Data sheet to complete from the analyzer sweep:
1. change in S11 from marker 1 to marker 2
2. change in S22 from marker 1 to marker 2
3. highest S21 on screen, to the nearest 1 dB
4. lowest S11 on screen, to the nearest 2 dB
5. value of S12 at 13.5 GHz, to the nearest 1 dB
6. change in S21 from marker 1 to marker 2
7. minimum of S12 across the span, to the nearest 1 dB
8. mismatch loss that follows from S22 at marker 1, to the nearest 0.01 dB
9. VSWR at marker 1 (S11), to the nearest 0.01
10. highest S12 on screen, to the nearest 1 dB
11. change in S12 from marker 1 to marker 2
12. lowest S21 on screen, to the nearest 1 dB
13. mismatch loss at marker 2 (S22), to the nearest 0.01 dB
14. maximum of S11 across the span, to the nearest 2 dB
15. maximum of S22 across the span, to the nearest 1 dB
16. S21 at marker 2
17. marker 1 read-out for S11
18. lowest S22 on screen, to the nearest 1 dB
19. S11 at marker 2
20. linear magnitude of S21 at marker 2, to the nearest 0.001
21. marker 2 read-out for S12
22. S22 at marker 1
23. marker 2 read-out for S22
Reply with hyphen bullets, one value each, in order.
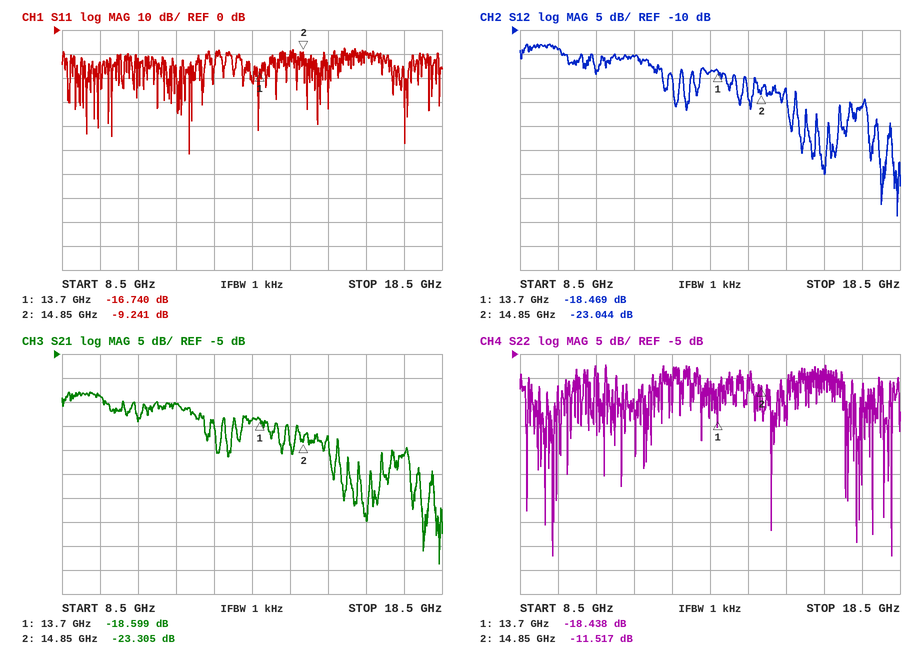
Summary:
- 7.499 dB
- 6.921 dB
- -13 dB
- -52 dB
- -19 dB
- -4.706 dB
- -49 dB
- 0.06 dB
- 1.34
- -13 dB
- -4.575 dB
- -49 dB
- 0.32 dB
- -8 dB
- -7 dB
- -23.305 dB
- -16.740 dB
- -47 dB
- -9.241 dB
- 0.068
- -23.044 dB
- -18.438 dB
- -11.517 dB
